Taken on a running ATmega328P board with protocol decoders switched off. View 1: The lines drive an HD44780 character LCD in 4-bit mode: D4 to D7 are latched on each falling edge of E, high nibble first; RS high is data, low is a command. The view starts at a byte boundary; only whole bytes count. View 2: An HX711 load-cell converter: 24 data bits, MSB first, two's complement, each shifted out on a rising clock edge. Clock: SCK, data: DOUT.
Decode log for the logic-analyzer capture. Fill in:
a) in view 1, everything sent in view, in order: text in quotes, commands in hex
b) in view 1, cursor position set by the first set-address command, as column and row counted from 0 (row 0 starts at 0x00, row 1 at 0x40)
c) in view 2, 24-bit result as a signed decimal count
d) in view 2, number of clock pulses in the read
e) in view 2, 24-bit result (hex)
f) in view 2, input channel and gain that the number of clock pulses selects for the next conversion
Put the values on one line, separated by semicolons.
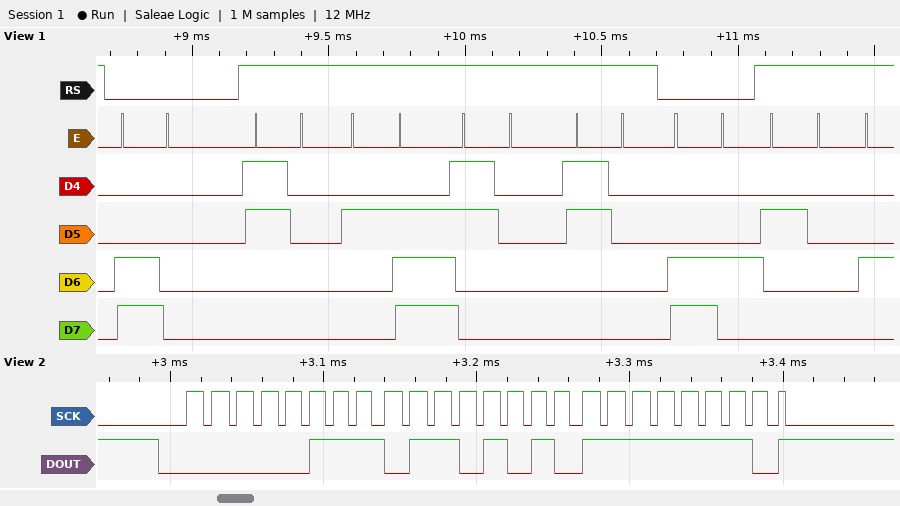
0xC0 "0.00" 0xC4 " "; column 0, row 1; 486142; 25; 0x076AFE; channel A, gain 128
